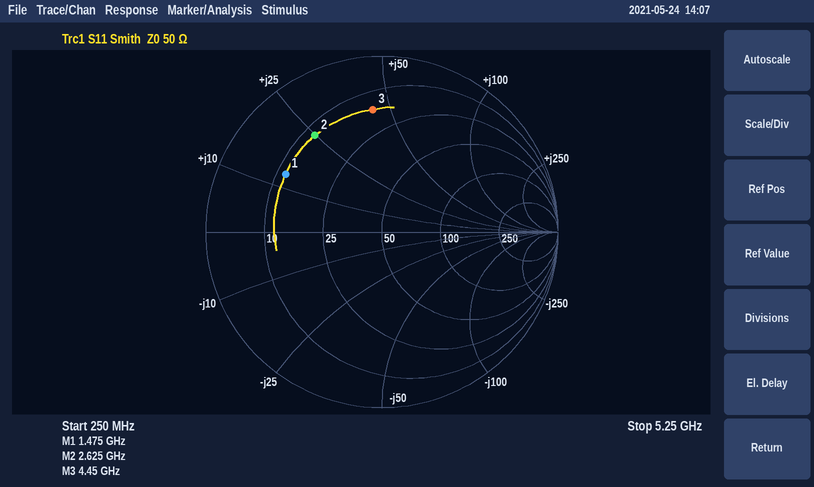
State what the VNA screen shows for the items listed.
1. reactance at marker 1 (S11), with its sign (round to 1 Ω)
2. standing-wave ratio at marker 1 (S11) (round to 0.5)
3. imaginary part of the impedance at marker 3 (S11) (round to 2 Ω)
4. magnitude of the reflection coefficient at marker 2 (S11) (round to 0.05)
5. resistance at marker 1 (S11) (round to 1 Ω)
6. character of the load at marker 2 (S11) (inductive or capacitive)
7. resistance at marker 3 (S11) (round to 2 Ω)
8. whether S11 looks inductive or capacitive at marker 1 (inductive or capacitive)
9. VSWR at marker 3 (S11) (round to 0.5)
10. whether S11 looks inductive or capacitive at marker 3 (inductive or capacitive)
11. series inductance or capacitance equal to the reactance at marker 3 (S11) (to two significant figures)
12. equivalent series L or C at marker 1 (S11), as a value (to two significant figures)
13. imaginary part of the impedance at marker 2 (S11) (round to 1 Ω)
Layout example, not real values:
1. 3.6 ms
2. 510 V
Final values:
1. +13 Ω
2. 4.5
3. +44 Ω
4. 0.65
5. 12 Ω
6. inductive
7. 16 Ω
8. inductive
9. 5.5
10. inductive
11. 1.6 nH
12. 1.4 nH
13. +25 Ω
